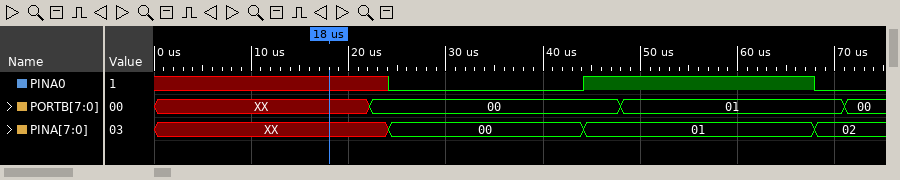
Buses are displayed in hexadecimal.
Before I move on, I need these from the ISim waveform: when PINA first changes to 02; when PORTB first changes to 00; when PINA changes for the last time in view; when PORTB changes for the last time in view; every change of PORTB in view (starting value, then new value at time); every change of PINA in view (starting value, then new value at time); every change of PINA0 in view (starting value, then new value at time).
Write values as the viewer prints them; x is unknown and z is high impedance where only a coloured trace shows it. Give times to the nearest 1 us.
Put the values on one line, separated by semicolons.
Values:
68 us; 22 us; 68 us; 71 us; XX, 00 at 22 us, 01 at 48 us, 00 at 71 us; XX, 00 at 24 us, 01 at 44 us, 02 at 68 us; x, 0 at 24 us, 1 at 44 us, 0 at 68 us
